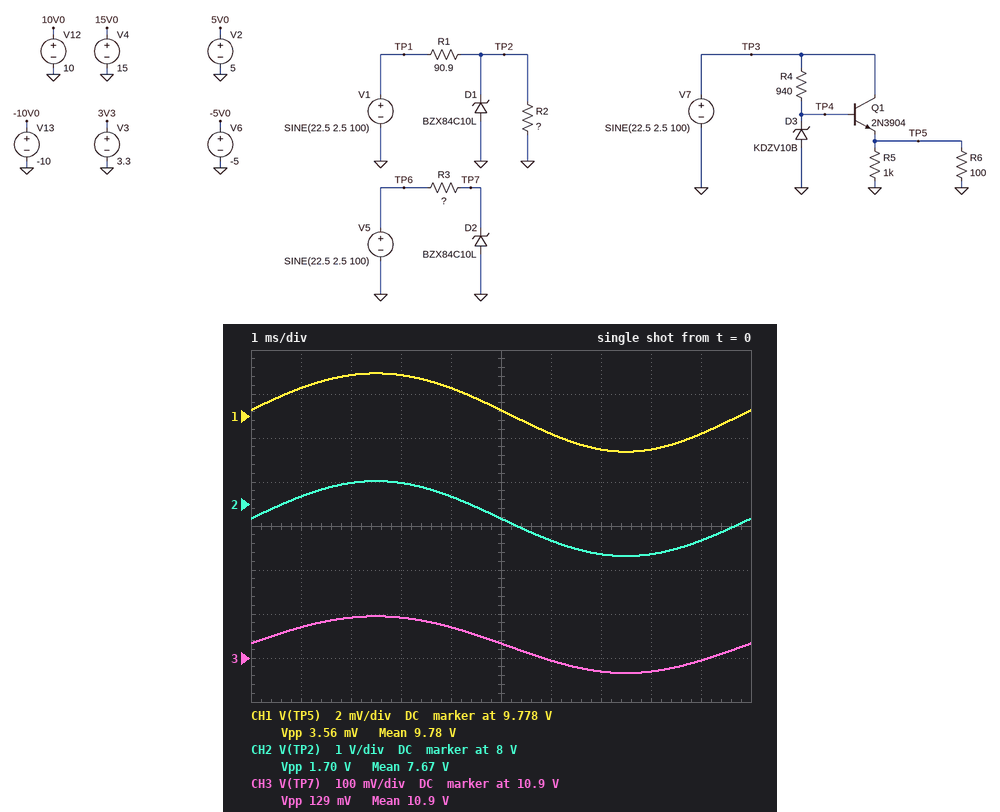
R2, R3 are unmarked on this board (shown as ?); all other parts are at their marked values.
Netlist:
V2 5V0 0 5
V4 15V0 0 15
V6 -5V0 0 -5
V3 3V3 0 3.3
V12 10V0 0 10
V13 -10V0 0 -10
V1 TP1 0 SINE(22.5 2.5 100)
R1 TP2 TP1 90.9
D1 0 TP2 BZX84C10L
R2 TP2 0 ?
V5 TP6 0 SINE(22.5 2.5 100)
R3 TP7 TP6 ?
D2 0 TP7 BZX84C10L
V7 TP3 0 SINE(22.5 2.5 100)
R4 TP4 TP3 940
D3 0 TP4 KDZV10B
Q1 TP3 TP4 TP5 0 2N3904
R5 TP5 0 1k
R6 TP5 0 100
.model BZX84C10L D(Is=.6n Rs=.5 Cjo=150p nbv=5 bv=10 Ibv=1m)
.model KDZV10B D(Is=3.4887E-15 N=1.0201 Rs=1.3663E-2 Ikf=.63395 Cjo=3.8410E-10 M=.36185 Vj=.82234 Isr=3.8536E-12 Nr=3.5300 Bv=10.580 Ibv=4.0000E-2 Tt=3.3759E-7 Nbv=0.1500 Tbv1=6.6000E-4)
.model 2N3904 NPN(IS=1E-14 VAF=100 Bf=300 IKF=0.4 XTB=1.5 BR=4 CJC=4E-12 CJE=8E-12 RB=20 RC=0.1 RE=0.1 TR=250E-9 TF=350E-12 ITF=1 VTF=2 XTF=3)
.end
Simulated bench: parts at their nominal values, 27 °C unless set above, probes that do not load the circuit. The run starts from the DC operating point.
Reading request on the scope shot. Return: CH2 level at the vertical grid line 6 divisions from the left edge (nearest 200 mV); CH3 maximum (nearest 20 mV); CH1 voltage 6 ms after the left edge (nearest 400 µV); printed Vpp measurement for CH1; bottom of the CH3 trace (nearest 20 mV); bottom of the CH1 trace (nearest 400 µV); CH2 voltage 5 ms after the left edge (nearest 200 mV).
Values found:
7.2 V
11.00 V
9.7772 V
3.56 mV
10.86 V
9.7764 V
7.6 V
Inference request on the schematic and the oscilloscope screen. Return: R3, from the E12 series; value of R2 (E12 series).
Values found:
33 Ω
47 Ω
